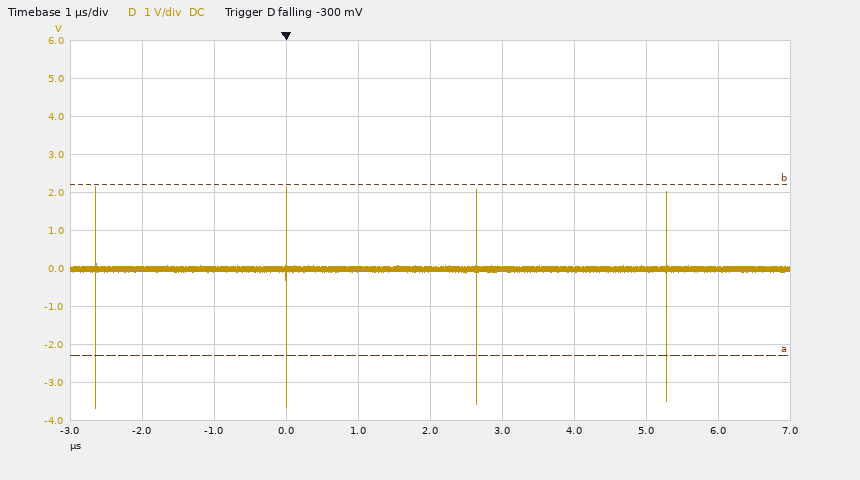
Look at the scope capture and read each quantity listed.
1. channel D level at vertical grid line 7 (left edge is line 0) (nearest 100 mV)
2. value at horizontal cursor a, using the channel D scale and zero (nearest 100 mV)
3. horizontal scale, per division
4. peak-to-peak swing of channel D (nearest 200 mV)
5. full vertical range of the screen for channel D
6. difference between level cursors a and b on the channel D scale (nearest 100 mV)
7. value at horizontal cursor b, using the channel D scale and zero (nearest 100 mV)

0.0 V
-2.3 V
1 µs
5.8 V
10 V
4.5 V
2.2 V
